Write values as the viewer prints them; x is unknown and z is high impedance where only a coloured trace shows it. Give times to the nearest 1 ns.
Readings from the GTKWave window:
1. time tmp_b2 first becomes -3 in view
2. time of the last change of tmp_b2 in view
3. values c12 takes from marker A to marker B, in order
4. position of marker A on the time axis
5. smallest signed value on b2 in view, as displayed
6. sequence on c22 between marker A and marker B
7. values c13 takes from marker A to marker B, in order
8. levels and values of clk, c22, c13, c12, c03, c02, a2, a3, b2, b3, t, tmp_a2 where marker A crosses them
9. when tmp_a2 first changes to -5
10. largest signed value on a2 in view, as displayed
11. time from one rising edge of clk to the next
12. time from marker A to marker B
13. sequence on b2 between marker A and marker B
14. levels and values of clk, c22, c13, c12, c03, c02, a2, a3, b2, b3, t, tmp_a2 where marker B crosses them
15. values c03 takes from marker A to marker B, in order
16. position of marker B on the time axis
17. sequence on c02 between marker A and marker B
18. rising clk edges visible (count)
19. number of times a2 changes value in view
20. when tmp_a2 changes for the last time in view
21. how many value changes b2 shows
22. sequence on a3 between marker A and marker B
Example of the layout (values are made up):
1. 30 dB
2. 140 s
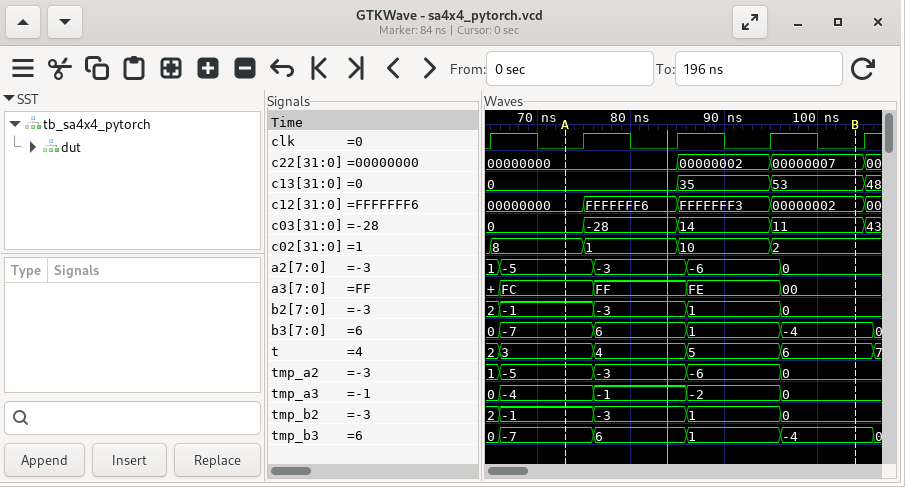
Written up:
1. 76 ns
2. 96 ns
3. 00000000, FFFFFFF6, FFFFFFF3, 00000002
4. 73 ns
5. -3
6. 00000000, 00000002, 00000007
7. 0, 35, 53
8. clk=0, c22=00000000, c13=0, c12=00000000, c03=0, c02=8, a2=-5, a3=FC, b2=-1, b3=-7, t=3, tmp_a2=-5
9. 66 ns
10. 1
11. 10 ns
12. 31 ns
13. -1, -3, 1, 0
14. clk=0, c22=00000007, c13=53, c12=00000002, c03=11, c02=2, a2=0, a3=00, b2=0, b3=-4, t=6, tmp_a2=0
15. 0, -28, 14, 11
16. 104 ns
17. 8, 1, 10, 2
18. 5
19. 4
20. 96 ns
21. 4
22. FC, FF, FE, 00
